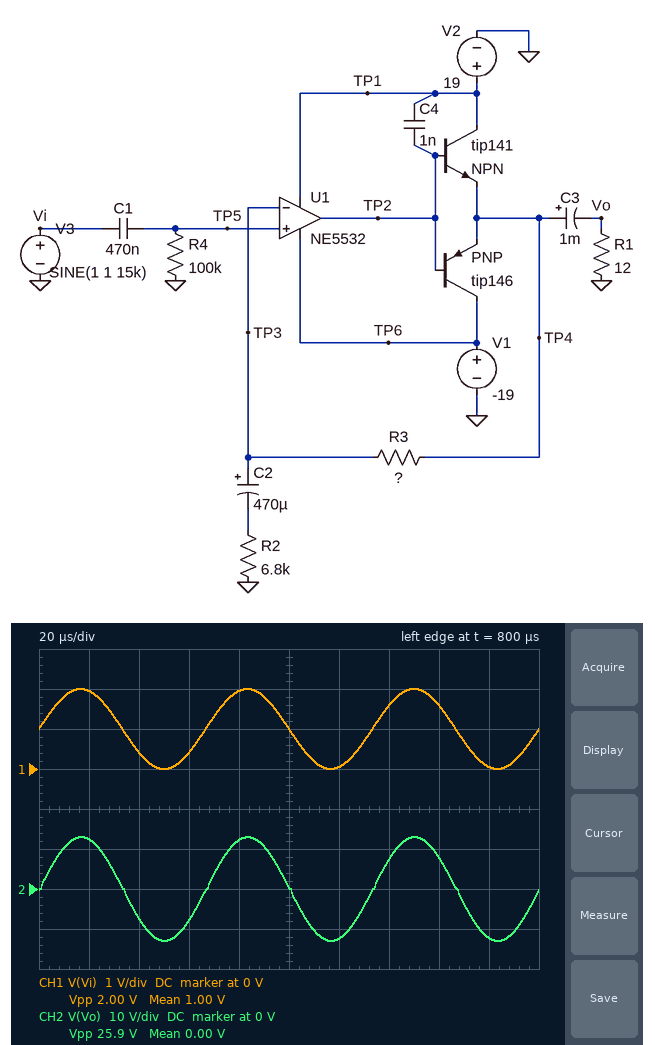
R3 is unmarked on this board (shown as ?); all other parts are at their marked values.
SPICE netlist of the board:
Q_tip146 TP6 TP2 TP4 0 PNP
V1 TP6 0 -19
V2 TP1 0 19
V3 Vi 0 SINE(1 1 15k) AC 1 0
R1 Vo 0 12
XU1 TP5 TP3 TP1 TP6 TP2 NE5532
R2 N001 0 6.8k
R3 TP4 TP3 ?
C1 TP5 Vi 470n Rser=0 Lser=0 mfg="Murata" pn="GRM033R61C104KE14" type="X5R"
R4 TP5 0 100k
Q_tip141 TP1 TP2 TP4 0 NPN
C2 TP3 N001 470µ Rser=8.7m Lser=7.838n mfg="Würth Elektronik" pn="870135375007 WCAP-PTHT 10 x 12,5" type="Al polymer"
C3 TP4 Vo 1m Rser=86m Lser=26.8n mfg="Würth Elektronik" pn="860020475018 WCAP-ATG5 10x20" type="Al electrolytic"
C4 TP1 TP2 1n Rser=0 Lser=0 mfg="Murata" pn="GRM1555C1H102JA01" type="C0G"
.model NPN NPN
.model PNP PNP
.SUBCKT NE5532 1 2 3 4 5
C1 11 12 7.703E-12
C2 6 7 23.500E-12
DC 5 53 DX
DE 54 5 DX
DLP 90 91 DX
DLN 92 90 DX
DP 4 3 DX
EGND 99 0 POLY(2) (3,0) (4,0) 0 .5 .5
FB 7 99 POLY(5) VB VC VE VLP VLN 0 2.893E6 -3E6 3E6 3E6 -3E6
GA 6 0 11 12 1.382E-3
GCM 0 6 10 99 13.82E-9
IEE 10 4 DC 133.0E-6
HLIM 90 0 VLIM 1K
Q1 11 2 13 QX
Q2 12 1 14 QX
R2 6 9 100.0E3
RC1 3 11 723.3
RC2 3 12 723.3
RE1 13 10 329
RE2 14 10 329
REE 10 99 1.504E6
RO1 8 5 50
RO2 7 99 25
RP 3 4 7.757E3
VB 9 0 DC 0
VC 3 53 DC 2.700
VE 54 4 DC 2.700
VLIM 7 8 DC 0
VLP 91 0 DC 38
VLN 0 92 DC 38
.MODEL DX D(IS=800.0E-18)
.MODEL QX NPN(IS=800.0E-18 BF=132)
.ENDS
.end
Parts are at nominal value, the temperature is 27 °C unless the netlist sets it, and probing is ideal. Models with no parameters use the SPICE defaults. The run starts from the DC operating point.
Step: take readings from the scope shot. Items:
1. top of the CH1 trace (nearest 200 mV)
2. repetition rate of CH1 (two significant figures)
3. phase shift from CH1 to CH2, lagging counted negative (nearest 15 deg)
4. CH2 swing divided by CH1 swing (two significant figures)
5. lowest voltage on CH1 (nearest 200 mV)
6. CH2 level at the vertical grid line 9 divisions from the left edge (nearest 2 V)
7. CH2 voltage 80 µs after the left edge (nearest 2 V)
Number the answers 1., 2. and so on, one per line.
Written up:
1. 2.0 V
2. 15 kHz
3. 0 deg
4. 13
5. 0 V
6. -12 V
7. 12 V
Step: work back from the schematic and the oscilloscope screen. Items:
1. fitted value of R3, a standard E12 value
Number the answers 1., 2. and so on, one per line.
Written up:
1. 82 kΩ
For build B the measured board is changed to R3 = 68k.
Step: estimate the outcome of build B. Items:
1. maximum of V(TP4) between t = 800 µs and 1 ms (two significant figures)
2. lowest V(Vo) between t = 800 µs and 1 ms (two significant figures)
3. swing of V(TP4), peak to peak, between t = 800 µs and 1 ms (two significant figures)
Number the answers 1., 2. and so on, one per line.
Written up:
1. 11 V
2. -11 V
3. 22 V
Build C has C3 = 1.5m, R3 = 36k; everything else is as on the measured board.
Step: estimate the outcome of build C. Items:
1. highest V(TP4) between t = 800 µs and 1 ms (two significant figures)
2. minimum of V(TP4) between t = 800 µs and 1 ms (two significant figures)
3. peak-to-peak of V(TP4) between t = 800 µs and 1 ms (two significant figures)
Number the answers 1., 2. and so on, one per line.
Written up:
1. 6.3 V
2. -6.3 V
3. 13 V
